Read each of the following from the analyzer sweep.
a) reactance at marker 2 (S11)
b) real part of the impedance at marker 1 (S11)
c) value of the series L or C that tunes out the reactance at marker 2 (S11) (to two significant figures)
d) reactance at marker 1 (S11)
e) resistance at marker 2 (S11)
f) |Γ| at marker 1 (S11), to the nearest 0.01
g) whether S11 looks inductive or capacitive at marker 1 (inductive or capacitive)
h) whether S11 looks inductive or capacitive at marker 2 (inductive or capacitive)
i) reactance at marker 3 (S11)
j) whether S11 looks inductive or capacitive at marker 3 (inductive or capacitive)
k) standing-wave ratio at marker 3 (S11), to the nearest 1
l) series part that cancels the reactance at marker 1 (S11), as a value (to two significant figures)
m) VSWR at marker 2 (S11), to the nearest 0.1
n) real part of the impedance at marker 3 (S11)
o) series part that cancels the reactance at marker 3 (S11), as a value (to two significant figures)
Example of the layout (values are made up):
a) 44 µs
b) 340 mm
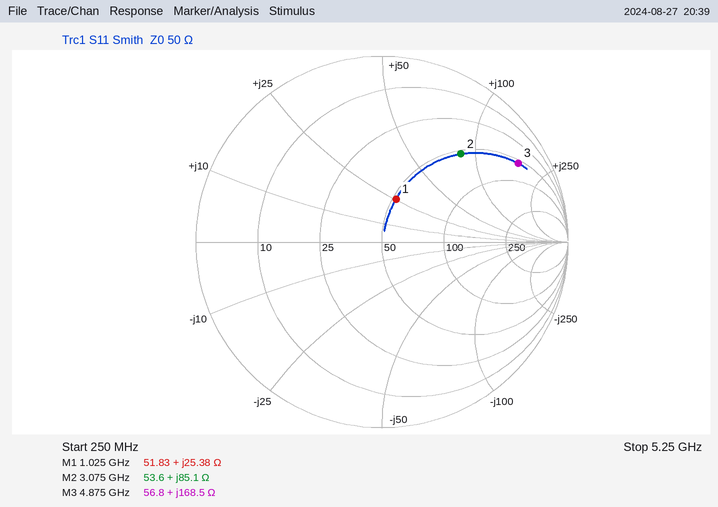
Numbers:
a) +85.1 Ω
b) 51.83 Ω
c) 610 fF
d) +25.38 Ω
e) 53.6 Ω
f) 0.24
g) inductive
h) inductive
i) +168.5 Ω
j) inductive
k) 12
l) 6.1 pF
m) 4.5
n) 56.8 Ω
o) 190 fF
